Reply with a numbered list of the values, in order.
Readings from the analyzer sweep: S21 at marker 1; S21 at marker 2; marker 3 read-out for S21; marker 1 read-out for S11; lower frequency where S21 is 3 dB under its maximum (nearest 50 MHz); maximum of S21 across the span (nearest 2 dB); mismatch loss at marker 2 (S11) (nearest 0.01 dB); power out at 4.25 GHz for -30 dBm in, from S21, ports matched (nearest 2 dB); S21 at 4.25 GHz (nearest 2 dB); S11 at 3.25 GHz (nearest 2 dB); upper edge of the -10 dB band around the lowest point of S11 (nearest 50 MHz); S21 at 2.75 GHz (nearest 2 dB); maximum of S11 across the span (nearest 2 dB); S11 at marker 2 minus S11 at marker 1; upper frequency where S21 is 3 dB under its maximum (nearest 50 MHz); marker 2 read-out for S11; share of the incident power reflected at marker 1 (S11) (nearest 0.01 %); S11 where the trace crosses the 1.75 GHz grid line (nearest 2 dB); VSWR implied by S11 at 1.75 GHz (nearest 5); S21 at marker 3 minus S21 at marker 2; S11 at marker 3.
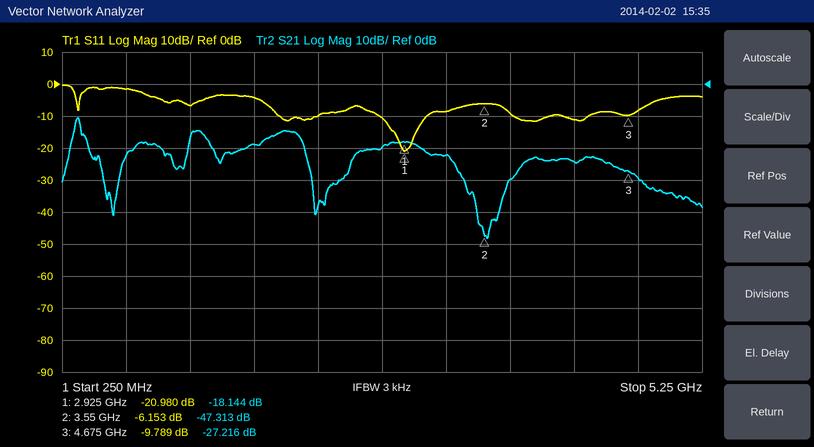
1. -18.144 dB
2. -47.313 dB
3. -27.216 dB
4. -20.980 dB
5. 350 MHz
6. -10 dB
7. 1.21 dB
8. -54 dBm
9. -24 dB
10. -8 dB
11. 3.10 GHz
12. -20 dB
13. 0 dB
14. 14.827 dB
15. 400 MHz
16. -6.153 dB
17. 0.80 %
18. -4 dB
19. 5
20. 20.097 dB
21. -9.789 dB
